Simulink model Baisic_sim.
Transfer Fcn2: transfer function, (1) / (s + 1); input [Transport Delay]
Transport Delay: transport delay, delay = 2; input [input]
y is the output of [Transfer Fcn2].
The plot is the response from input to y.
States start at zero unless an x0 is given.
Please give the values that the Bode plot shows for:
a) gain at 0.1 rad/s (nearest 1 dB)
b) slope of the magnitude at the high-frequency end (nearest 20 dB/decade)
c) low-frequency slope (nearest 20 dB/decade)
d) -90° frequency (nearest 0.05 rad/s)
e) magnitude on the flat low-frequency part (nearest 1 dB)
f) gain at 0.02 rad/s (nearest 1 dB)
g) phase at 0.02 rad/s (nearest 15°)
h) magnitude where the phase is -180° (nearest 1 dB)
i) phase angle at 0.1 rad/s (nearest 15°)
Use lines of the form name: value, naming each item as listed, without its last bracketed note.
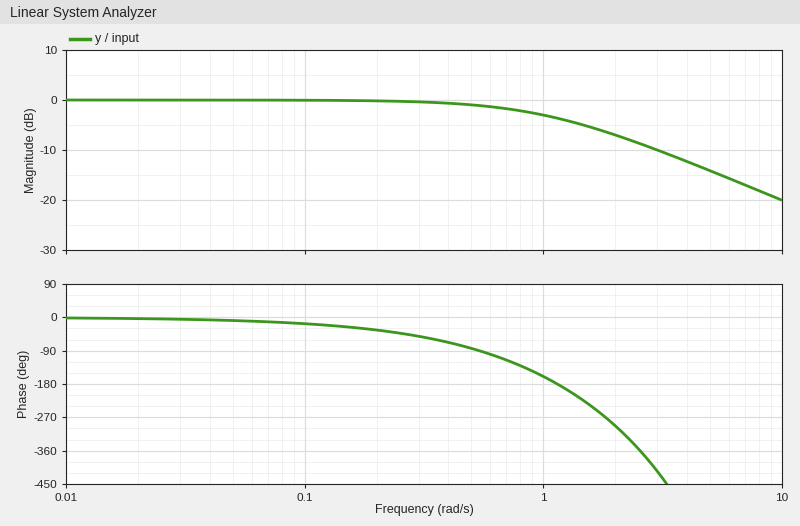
gain at 0.1 rad/s: 0 dB
slope of the magnitude at the high-frequency end: -20 dB/decade
low-frequency slope: 0 dB/decade
-90° frequency: 0.55 rad/s
magnitude on the flat low-frequency part: 0 dB
gain at 0.02 rad/s: 0 dB
phase at 0.02 rad/s: 0°
magnitude where the phase is -180°: -4 dB
phase angle at 0.1 rad/s: -15°
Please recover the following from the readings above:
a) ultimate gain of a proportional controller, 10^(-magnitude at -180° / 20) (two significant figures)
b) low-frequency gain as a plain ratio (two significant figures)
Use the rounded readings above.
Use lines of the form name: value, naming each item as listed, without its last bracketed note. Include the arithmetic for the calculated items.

ultimate gain of a proportional controller, 10^(-magnitude at -180° / 20): 10^(4 / 20) = 1.6
low-frequency gain as a plain ratio: 10^(0 / 20) = 1.0
